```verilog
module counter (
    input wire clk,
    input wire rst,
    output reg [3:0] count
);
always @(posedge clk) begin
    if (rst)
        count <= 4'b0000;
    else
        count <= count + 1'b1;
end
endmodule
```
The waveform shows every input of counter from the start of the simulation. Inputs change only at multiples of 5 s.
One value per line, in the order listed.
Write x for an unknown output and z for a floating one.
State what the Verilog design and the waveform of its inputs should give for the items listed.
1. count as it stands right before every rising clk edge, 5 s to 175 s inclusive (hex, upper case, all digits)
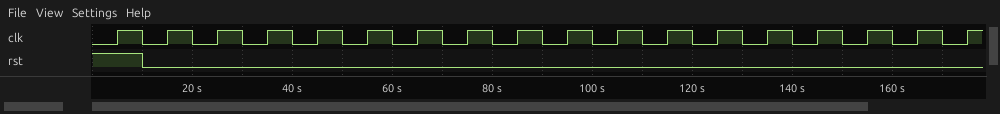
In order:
x, 0, 1, 2, 3, 4, 5, 6, 7, 8, 9, A, B, C, D, E, F, 0
